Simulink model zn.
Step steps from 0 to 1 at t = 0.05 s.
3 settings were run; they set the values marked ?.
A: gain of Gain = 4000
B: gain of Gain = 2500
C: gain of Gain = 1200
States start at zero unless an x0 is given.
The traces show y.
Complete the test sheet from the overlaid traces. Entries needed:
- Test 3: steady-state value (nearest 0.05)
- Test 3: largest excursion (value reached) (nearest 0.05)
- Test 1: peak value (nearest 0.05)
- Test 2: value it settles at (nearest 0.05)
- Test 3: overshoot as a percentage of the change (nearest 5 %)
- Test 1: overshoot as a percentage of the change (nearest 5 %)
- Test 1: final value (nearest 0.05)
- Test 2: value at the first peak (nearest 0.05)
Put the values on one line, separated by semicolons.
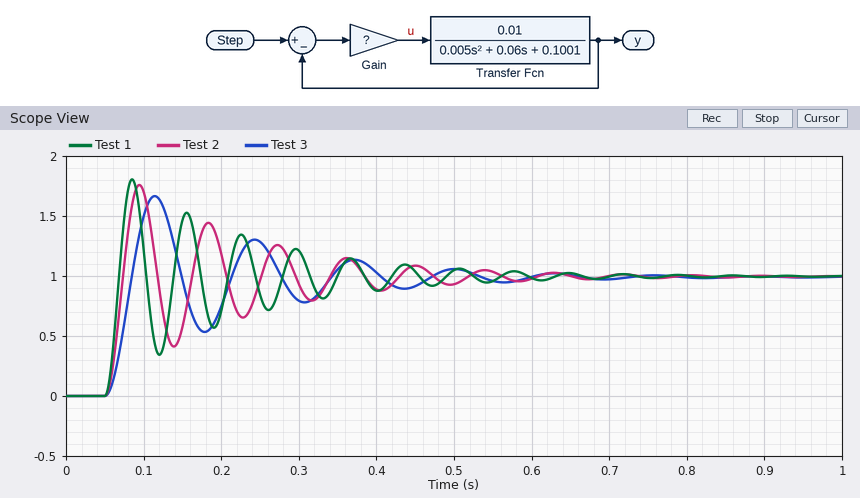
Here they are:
1.00; 1.65; 1.80; 1.00; 70 %; 80 %; 1.00; 1.75
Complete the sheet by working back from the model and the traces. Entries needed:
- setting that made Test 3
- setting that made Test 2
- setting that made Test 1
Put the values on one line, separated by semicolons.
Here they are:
C; B; A
